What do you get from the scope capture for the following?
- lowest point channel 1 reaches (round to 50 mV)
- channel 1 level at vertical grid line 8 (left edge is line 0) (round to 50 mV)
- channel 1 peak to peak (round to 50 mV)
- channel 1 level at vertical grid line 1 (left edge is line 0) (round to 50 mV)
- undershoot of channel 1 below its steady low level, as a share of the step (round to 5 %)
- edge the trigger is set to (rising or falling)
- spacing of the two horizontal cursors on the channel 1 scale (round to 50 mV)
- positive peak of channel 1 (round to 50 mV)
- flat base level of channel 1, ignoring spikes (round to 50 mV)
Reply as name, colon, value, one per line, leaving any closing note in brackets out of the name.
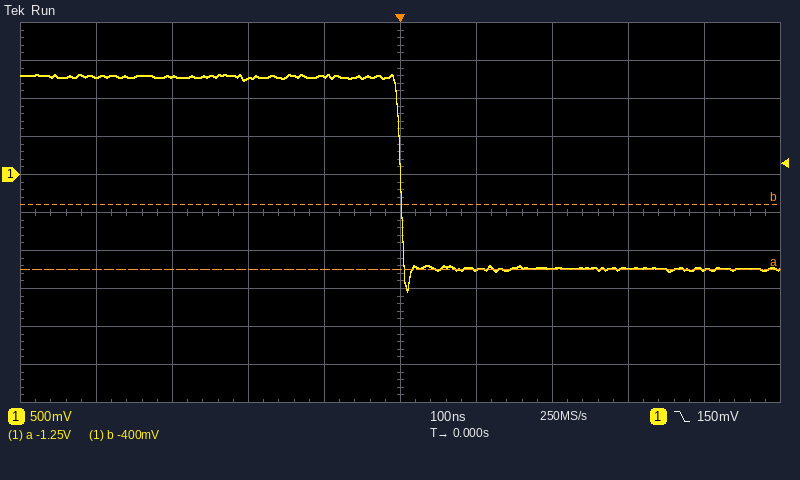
lowest point channel 1 reaches: -1.55 V
channel 1 level at vertical grid line 8 (left edge is line 0): -1.25 V
channel 1 peak to peak: 2.85 V
channel 1 level at vertical grid line 1 (left edge is line 0): 1.30 V
undershoot of channel 1 below its steady low level, as a share of the step: 10 %
edge the trigger is set to: falling
spacing of the two horizontal cursors on the channel 1 scale: 850 mV
positive peak of channel 1: 1.30 V
flat base level of channel 1, ignoring spikes: -1.25 V
